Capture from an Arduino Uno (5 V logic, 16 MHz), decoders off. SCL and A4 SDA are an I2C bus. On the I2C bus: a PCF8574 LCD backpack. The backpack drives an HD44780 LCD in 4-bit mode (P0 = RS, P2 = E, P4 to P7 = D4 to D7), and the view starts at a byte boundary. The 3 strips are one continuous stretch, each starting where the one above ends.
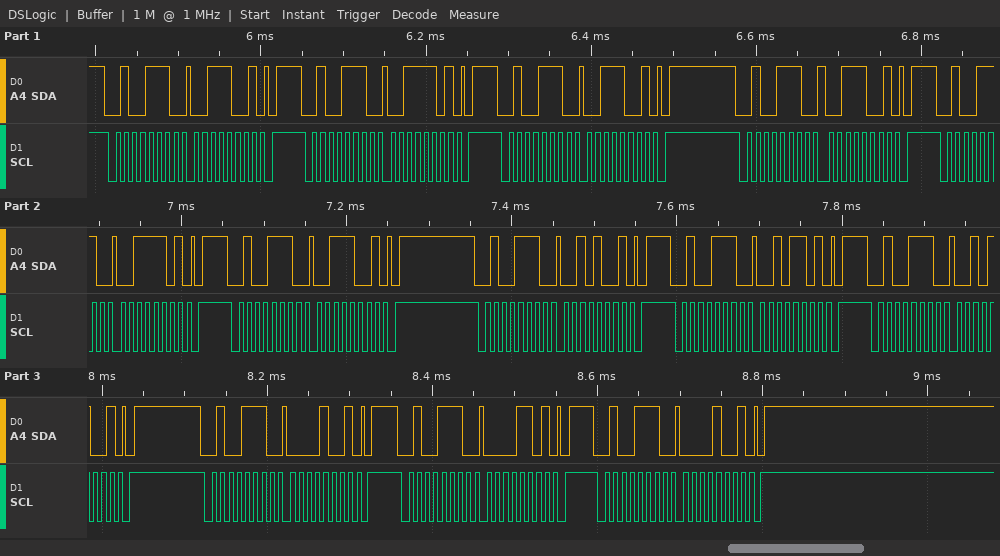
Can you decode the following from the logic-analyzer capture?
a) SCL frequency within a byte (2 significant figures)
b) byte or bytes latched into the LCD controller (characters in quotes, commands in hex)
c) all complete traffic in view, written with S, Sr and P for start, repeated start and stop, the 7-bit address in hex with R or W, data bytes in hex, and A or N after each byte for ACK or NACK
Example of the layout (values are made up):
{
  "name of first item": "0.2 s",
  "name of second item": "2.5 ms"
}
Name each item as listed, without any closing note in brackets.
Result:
{
  "SCL frequency within a byte": "100 kHz",
  "byte or bytes latched into the LCD controller": "'3' ' '",
  "all complete traffic in view, written with S, Sr and P for start, repeated start and stop, the 7-bit address in hex with R or W, data bytes in hex, and A or N after each byte for ACK or NACK": "S 27W A 39 A P S 27W A 3D A P S 27W A 39 A P S 27W A 39 A P S 27W A 3D A P S 27W A 39 A P S 27W A 29 A P S 27W A 2D A P S 27W A 29 A P S 27W A 09 A P S 27W A 0D A P S 27W A 09 A P"
}
